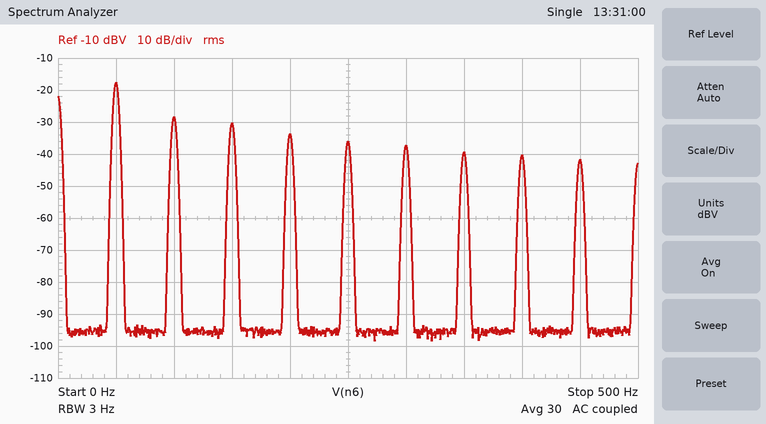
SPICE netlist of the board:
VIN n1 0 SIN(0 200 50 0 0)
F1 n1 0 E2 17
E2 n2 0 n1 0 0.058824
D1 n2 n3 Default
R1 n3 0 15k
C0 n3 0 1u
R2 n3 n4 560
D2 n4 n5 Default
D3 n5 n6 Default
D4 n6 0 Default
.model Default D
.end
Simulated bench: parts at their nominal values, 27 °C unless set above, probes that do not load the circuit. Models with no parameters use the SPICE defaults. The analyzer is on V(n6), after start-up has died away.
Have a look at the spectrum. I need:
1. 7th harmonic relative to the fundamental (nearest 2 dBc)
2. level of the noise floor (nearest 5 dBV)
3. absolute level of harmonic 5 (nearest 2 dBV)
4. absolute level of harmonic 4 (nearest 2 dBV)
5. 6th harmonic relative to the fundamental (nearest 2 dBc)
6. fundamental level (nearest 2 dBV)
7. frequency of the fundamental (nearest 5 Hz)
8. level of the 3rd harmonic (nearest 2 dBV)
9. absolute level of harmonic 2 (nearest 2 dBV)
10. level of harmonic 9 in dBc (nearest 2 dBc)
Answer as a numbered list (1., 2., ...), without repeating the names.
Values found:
1. -22 dBc
2. -95 dBV
3. -36 dBV
4. -34 dBV
5. -20 dBc
6. -18 dBV
7. 50 Hz
8. -30 dBV
9. -28 dBV
10. -24 dBc
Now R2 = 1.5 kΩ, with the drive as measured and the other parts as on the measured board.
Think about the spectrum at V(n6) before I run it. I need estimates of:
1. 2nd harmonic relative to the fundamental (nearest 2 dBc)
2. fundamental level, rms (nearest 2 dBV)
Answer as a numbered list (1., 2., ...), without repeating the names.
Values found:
1. -8 dBc
2. -20 dBV
